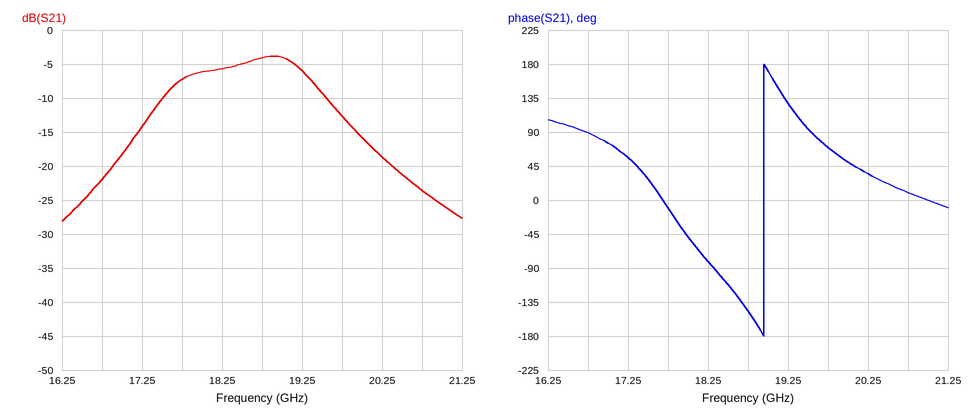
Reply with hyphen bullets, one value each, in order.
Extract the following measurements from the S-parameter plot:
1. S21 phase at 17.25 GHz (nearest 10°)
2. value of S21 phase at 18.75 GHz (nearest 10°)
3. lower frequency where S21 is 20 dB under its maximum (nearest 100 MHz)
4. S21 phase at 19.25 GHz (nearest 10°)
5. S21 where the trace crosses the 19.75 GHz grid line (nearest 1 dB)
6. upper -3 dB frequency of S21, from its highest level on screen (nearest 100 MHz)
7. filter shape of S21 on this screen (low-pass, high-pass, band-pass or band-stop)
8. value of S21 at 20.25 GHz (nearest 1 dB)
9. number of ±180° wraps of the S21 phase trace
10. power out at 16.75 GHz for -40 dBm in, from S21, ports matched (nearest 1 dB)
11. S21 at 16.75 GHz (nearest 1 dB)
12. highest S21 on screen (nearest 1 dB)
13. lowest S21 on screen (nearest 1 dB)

- 60°
- -150°
- 16.6 GHz
- 130°
- -13 dB
- 19.3 GHz
- band-pass
- -19 dB
- 1
- -62 dBm
- -22 dB
- -4 dB
- -28 dB
